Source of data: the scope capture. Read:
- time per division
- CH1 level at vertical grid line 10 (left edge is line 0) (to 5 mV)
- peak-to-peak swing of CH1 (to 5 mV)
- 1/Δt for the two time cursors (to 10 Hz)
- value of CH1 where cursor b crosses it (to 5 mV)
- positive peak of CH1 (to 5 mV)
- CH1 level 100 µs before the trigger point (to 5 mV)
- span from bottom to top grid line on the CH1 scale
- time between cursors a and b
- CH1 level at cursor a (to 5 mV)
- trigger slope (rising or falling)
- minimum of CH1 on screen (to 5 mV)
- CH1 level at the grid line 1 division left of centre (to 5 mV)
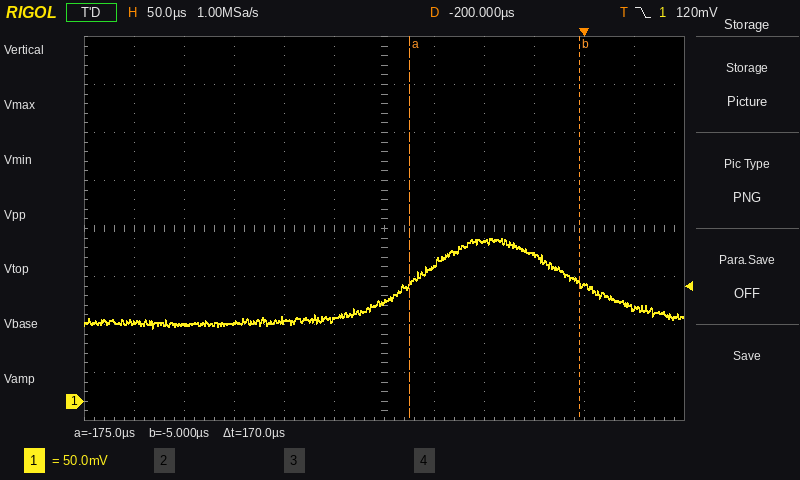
50 µs
120 mV
95 mV
5.88 kHz
125 mV
170 mV
165 mV
400 mV
170 µs
120 mV
falling
75 mV
85 mV
